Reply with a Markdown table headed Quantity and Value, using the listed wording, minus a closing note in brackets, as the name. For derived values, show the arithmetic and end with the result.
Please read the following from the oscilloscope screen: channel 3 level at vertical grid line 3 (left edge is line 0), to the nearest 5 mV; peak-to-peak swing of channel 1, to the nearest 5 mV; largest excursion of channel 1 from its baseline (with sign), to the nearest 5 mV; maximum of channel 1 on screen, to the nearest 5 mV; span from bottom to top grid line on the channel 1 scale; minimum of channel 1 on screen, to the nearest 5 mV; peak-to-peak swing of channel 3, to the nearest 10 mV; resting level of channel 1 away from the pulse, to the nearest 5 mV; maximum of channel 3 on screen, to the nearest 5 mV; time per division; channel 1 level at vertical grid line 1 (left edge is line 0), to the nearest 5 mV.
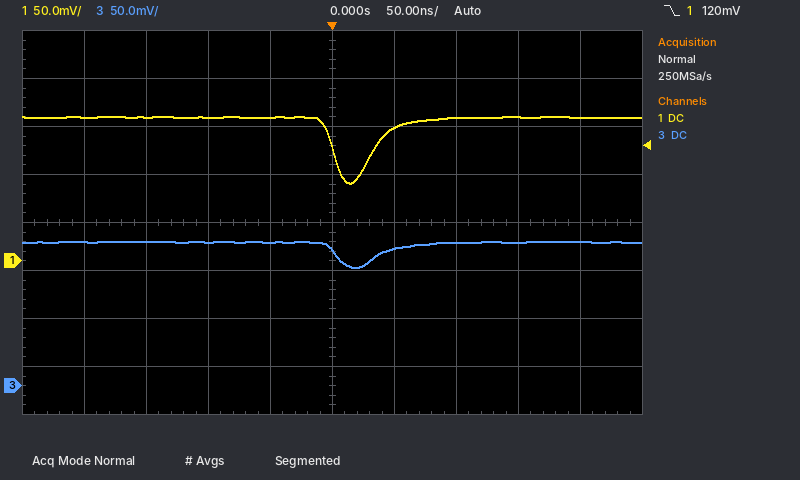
| Quantity | Value |
|---|---|
| channel 3 level at vertical grid line 3 (left edge is line 0), to the nearest 5 mV | 150 mV |
| peak-to-peak swing of channel 1, to the nearest 5 mV | 150 mV − (80 mV) = 70 mV |
| largest excursion of channel 1 from its baseline (with sign), to the nearest 5 mV | 80 mV − (150 mV) = -70 mV |
| maximum of channel 1 on screen, to the nearest 5 mV | 150 mV |
| span from bottom to top grid line on the channel 1 scale | 400 mV |
| minimum of channel 1 on screen, to the nearest 5 mV | 80 mV |
| peak-to-peak swing of channel 3, to the nearest 10 mV | 30 mV |
| resting level of channel 1 away from the pulse, to the nearest 5 mV | 150 mV |
| maximum of channel 3 on screen, to the nearest 5 mV | 150 mV |
| time per division | 50 ns |
| channel 1 level at vertical grid line 1 (left edge is line 0), to the nearest 5 mV | 150 mV |
